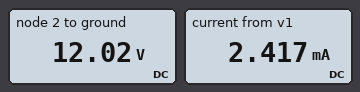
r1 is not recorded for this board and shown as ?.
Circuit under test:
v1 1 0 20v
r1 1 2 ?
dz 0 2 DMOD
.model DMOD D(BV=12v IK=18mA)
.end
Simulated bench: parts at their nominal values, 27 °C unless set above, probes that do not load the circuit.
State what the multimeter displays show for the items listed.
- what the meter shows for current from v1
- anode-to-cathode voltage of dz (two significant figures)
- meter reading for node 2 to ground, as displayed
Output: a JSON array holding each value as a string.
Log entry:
["2.417 mA", "-12 V", "12.02 V"]
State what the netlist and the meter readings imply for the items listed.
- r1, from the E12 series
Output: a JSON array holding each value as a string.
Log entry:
["3.3 kΩ"]
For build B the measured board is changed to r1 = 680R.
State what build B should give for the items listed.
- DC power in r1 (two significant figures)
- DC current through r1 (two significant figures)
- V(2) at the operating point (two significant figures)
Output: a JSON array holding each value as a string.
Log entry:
["93 mW", "12 mA", "12 V"]
